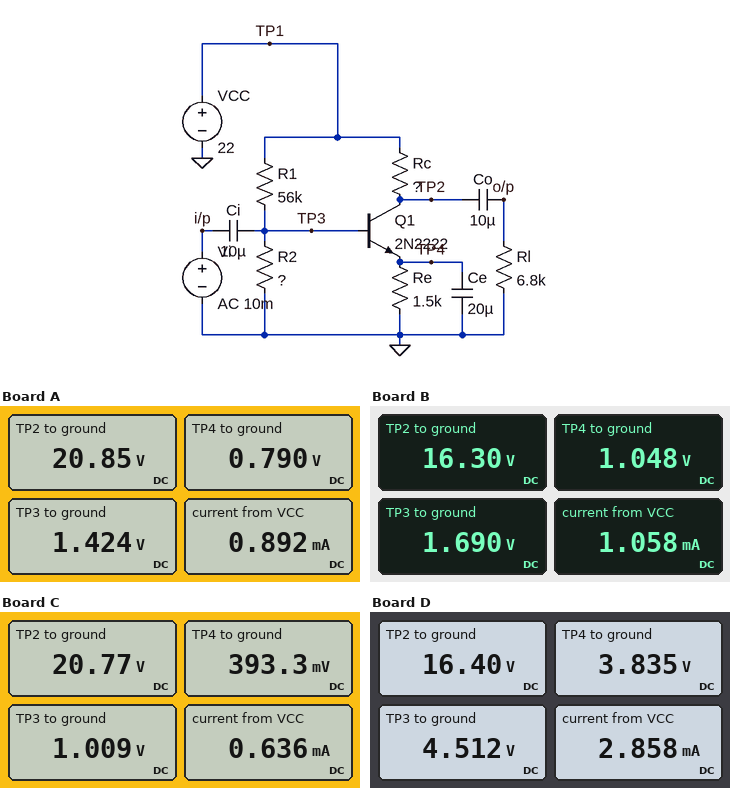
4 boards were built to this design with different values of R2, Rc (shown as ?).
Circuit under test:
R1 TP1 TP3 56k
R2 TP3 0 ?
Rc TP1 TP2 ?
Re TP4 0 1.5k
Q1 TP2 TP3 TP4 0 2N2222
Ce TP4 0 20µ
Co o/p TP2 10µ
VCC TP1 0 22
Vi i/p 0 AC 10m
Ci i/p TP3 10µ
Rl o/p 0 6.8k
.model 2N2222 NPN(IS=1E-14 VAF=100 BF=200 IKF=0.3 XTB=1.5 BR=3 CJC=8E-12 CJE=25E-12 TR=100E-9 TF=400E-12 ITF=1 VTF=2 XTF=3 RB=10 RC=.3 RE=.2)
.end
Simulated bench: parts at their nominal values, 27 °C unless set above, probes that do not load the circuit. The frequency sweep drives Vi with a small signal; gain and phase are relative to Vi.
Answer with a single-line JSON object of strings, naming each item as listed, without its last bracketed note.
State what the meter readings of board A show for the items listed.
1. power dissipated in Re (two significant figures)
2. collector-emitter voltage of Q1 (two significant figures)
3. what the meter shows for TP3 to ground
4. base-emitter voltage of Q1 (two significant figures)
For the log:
{"power dissipated in Re": "420 µW", "collector-emitter voltage of Q1": "20 V", "what the meter shows for TP3 to ground": "1.424 V", "base-emitter voltage of Q1": "630 mV"}
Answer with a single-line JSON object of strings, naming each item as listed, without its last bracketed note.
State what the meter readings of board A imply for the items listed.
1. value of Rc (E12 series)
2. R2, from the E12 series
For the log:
{"value of Rc": "2.2 kΩ", "R2, from the E12 series": "3.9 kΩ"}
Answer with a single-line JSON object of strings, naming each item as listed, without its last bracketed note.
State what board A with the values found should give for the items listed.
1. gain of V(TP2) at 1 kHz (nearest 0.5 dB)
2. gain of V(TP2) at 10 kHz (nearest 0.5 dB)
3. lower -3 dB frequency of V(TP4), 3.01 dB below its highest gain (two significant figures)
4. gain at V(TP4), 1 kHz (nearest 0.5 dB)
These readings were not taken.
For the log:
{"gain of V(TP2) at 1 kHz": "30.5 dB", "gain of V(TP2) at 10 kHz": "30.5 dB", "lower -3 dB frequency of V(TP4), 3.01 dB below its highest gain": "4.2 Hz", "gain at V(TP4), 1 kHz": "-16.0 dB"}
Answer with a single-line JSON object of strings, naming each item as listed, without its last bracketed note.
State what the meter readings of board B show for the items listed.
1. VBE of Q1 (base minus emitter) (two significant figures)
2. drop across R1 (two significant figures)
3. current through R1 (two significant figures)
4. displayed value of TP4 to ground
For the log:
{"VBE of Q1 (base minus emitter)": "640 mV", "drop across R1": "20 V", "current through R1": "360 µA", "displayed value of TP4 to ground": "1.048 V"}
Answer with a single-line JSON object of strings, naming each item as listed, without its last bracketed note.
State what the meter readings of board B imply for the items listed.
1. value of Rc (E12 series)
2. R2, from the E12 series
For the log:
{"value of Rc": "8.2 kΩ", "R2, from the E12 series": "4.7 kΩ"}
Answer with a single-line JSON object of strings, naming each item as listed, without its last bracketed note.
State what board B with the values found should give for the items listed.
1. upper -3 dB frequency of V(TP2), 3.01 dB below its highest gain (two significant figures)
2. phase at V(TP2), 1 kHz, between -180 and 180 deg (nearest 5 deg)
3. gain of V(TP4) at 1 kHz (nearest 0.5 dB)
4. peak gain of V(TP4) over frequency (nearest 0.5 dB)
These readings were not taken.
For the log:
{"upper -3 dB frequency of V(TP2), 3.01 dB below its highest gain": "12 MHz", "phase at V(TP2), 1 kHz, between -180 and 180 deg": "-170 deg", "gain of V(TP4) at 1 kHz": "-14.0 dB", "peak gain of V(TP4) over frequency": "-0.5 dB"}
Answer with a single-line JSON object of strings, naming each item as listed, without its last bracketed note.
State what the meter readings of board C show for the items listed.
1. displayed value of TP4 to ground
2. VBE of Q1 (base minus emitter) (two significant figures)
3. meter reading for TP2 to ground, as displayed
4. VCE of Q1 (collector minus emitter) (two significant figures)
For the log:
{"displayed value of TP4 to ground": "393.3 mV", "VBE of Q1 (base minus emitter)": "620 mV", "meter reading for TP2 to ground, as displayed": "20.77 V", "VCE of Q1 (collector minus emitter)": "20 V"}
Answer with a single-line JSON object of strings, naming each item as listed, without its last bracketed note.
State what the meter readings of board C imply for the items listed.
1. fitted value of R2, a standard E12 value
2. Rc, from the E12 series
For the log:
{"fitted value of R2, a standard E12 value": "2.7 kΩ", "Rc, from the E12 series": "4.7 kΩ"}
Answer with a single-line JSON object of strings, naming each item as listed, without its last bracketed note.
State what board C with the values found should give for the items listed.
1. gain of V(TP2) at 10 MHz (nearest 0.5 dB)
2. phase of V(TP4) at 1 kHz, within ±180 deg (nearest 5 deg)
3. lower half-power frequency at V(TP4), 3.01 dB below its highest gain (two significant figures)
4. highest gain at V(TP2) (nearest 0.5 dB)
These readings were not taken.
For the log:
{"gain of V(TP2) at 10 MHz": "28.0 dB", "phase of V(TP4) at 1 kHz, within ±180 deg": "-85 deg", "lower half-power frequency at V(TP4), 3.01 dB below its highest gain": "5.4 Hz", "highest gain at V(TP2)": "29.0 dB"}
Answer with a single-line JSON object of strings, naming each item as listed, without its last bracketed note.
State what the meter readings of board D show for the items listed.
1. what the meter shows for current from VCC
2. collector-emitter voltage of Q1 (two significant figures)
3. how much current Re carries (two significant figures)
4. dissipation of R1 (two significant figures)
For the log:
{"what the meter shows for current from VCC": "2.858 mA", "collector-emitter voltage of Q1": "13 V", "how much current Re carries": "2.6 mA", "dissipation of R1": "5.5 mW"}
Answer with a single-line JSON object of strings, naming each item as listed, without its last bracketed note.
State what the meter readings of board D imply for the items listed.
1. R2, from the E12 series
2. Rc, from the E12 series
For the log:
{"R2, from the E12 series": "15 kΩ", "Rc, from the E12 series": "2.2 kΩ"}
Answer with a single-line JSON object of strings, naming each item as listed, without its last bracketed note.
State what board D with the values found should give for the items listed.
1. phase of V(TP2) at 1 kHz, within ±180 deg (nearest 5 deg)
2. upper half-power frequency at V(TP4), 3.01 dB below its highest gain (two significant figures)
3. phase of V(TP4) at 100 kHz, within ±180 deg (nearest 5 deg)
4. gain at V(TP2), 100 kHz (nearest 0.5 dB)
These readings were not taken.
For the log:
{"phase of V(TP2) at 1 kHz, within ±180 deg": "-145 deg", "upper half-power frequency at V(TP4), 3.01 dB below its highest gain": "750 Hz", "phase of V(TP4) at 100 kHz, within ±180 deg": "-90 deg", "gain at V(TP2), 100 kHz": "43.5 dB"}
